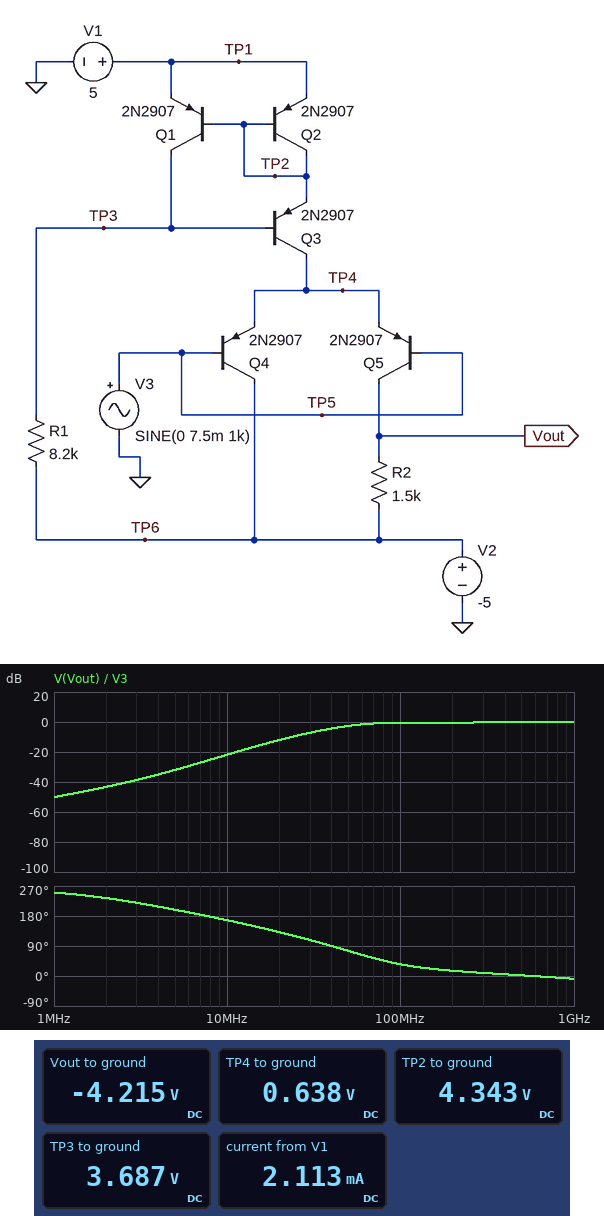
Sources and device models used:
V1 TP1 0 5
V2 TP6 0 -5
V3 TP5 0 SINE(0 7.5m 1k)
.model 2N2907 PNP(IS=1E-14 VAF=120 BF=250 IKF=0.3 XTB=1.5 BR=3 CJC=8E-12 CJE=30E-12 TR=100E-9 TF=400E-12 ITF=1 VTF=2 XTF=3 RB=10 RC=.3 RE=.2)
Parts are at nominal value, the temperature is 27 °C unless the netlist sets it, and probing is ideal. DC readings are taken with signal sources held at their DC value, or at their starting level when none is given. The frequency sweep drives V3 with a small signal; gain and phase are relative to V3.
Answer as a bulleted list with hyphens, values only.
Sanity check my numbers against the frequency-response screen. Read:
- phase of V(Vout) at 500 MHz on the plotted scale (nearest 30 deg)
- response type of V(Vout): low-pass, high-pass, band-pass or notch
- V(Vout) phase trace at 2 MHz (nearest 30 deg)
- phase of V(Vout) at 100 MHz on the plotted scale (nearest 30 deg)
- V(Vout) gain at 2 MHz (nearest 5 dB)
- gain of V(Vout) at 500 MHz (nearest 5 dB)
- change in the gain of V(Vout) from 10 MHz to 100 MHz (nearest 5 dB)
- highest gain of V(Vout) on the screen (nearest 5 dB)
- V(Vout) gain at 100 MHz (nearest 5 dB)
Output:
- 0 deg
- high-pass
- 240 deg
- 30 deg
- -45 dB
- 0 dB
- 20 dB
- 0 dB
- 0 dB
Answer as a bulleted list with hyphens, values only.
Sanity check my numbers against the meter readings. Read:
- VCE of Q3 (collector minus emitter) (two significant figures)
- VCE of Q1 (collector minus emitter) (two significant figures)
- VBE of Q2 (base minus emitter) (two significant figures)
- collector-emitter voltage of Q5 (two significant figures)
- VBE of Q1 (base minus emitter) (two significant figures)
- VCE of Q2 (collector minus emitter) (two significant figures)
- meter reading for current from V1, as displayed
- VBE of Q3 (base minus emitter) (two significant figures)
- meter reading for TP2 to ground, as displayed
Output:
- -3.7 V
- -1.3 V
- -660 mV
- -4.9 V
- -660 mV
- -660 mV
- 2.113 mA
- -660 mV
- 4.343 V
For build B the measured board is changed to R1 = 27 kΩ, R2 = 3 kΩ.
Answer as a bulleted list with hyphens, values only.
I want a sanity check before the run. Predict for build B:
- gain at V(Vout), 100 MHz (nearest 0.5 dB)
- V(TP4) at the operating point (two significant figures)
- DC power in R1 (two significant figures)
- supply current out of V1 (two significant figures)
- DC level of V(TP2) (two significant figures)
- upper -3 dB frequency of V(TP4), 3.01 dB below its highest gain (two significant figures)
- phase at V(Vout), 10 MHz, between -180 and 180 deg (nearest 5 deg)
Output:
- 0 dB
- 610 mV
- 2.8 mW
- 650 µA
- 4.4 V
- 3.5 GHz
- 125 deg
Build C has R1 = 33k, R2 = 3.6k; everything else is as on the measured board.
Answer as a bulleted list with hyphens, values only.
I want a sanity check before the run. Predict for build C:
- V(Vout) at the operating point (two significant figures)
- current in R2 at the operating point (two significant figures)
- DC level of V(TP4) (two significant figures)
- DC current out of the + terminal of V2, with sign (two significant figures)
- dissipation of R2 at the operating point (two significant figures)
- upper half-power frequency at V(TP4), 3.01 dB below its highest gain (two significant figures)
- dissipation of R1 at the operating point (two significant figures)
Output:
- -4.5 V
- 130 µA
- 600 mV
- -530 µA
- 62 µW
- 3.5 GHz
- 2.3 mW
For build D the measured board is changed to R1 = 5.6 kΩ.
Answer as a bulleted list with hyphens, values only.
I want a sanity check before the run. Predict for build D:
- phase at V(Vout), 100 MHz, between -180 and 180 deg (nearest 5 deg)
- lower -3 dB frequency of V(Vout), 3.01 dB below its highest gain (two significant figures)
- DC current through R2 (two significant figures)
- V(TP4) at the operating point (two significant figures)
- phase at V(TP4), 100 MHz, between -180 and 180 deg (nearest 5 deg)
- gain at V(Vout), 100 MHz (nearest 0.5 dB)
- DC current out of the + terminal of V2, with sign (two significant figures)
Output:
- 45 deg
- 61 MHz
- 760 µA
- 650 mV
- -5 deg
- -1.0 dB
- -3.1 mA
